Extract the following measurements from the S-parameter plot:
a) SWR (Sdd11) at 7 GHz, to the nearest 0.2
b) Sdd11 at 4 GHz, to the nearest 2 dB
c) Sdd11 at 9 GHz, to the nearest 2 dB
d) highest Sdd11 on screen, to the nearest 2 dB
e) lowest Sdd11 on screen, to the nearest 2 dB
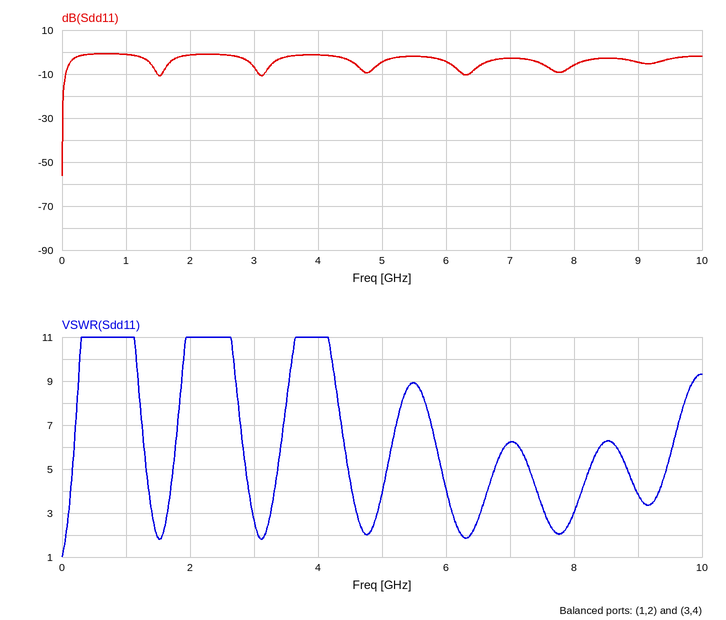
6.2
-2 dB
-4 dB
0 dB
-56 dB
